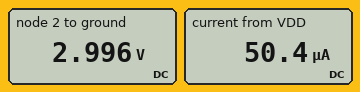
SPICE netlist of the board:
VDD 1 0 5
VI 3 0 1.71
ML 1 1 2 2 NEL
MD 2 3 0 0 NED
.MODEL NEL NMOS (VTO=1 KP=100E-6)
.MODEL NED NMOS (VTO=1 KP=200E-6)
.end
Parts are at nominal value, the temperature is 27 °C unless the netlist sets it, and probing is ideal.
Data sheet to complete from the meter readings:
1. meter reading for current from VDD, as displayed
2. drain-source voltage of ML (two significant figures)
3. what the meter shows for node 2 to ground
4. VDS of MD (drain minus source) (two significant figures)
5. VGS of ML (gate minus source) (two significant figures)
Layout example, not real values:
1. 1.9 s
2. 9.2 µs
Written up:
1. 50.4 µA
2. 2.0 V
3. 2.996 V
4. 3.0 V
5. 2.0 V
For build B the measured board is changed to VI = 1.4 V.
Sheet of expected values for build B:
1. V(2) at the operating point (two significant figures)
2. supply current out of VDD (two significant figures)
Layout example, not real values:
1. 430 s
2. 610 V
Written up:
1. 3.4 V
2. 16 µA
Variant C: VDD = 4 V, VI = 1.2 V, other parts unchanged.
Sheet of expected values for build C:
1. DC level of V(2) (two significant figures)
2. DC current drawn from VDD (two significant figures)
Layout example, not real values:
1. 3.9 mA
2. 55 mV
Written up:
1. 2.7 V
2. 4.0 µA
